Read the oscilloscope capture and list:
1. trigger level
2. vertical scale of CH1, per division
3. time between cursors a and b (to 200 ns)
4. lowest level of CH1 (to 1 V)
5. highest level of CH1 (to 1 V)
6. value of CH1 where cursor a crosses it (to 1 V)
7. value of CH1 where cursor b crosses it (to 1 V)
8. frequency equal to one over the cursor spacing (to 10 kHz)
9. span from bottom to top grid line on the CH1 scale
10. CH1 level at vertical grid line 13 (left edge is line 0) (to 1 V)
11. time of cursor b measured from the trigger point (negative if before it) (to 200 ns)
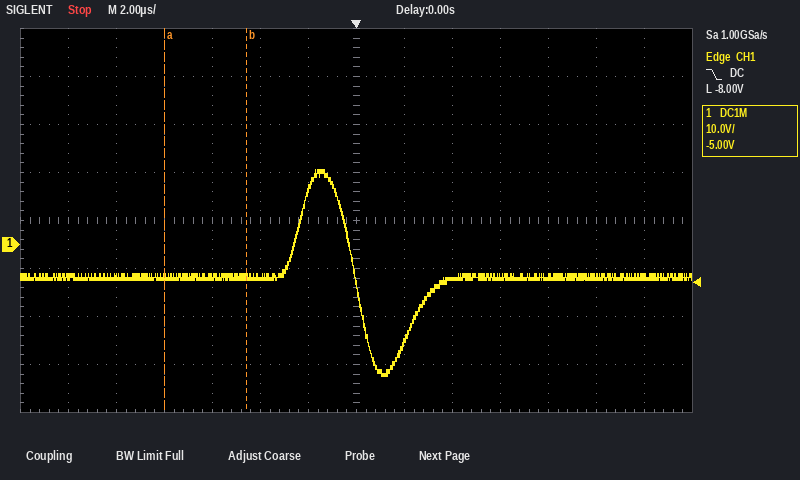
-8.00 V
10 V
3.4 µs
-28 V
16 V
-7 V
-7 V
290 kHz
80 V
-7 V
-4.6 µs
